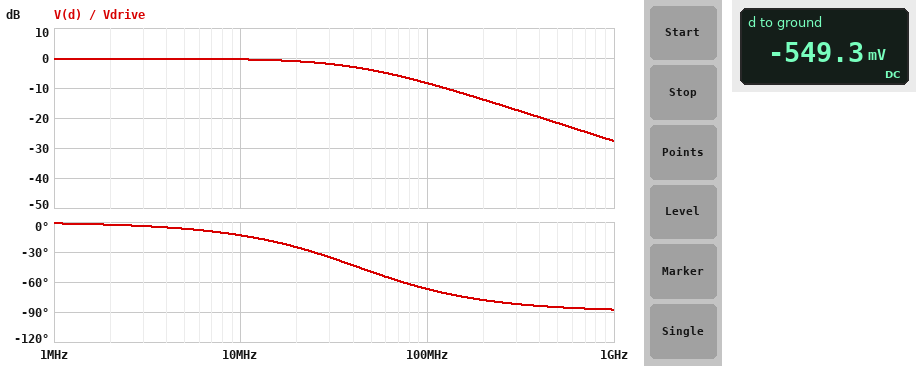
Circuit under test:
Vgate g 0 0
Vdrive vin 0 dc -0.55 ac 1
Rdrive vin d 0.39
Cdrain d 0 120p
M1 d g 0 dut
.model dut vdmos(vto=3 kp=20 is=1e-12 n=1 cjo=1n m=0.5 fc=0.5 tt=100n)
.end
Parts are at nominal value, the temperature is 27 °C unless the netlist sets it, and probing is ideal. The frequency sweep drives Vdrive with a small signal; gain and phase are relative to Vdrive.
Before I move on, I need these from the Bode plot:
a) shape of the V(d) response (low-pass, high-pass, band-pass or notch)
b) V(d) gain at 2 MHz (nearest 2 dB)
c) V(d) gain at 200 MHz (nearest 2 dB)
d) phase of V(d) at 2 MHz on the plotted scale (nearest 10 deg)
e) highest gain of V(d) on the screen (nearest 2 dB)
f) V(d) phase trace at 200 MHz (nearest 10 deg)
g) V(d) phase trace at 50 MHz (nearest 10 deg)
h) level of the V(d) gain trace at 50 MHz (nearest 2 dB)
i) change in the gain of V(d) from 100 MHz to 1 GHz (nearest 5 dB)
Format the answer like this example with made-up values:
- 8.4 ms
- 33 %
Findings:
- low-pass
- 0 dB
- -14 dB
- 0 deg
- 0 dB
- -80 deg
- -50 deg
- -4 dB
- -20 dB
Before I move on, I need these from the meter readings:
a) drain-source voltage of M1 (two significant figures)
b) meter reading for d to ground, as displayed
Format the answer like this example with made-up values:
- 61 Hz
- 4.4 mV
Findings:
- -550 mV
- -549.3 mV
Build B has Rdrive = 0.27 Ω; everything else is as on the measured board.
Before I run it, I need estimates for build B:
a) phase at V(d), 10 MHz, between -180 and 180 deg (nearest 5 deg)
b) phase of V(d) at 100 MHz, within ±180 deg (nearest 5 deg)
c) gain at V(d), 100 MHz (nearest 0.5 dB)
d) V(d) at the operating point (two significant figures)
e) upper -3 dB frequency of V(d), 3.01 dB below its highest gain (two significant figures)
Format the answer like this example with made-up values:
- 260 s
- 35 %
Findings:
- -10 deg
- -60 deg
- -6.0 dB
- -550 mV
- 60 MHz
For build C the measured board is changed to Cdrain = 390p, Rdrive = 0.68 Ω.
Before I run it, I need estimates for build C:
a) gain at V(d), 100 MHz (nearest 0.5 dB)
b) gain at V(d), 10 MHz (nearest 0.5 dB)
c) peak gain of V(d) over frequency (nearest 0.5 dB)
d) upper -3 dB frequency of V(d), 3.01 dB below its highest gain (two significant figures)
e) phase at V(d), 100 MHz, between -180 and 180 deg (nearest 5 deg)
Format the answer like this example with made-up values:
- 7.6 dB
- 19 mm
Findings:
- -13.0 dB
- -1.0 dB
- -0.5 dB
- 24 MHz
- -75 deg
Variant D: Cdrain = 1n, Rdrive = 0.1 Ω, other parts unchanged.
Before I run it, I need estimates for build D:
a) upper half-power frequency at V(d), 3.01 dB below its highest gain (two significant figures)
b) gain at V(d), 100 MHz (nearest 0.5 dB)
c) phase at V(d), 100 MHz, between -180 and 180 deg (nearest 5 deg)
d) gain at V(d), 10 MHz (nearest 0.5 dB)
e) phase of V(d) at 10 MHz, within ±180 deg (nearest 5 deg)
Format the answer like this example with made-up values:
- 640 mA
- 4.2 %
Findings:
- 150 MHz
- -1.5 dB
- -35 deg
- 0 dB
- -5 deg
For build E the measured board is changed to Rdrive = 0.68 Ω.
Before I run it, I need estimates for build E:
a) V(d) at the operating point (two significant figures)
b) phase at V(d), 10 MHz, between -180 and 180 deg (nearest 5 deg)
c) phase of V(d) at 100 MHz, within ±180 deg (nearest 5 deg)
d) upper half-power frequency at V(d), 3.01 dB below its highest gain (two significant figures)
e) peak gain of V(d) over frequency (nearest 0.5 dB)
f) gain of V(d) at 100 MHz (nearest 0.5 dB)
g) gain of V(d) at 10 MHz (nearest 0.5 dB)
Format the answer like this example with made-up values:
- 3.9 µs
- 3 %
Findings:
- -550 mV
- -20 deg
- -75 deg
- 25 MHz
- -0.5 dB
- -12.5 dB
- -1.0 dB
